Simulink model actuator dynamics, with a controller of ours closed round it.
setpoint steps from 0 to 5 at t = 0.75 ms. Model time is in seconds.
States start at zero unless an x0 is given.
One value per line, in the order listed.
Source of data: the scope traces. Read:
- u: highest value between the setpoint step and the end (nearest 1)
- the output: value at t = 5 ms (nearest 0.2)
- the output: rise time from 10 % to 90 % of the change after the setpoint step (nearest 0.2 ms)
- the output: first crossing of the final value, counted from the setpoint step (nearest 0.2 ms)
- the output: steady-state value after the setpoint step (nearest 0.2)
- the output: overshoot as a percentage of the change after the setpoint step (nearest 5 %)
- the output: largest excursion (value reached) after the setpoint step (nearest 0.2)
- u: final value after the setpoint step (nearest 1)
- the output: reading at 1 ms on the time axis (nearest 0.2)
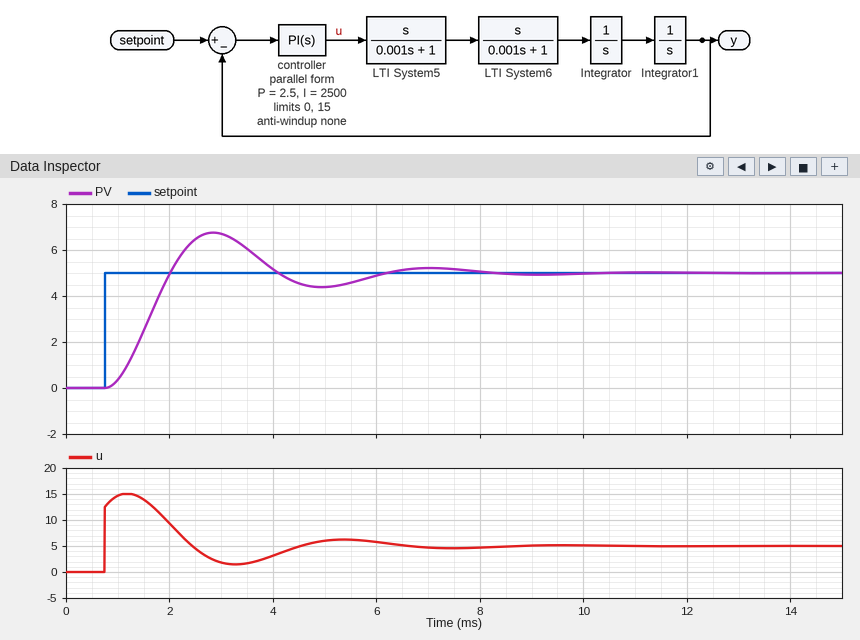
15
4.4
0.8 ms
1.2 ms
5.0
35 %
6.8
5
0.4
